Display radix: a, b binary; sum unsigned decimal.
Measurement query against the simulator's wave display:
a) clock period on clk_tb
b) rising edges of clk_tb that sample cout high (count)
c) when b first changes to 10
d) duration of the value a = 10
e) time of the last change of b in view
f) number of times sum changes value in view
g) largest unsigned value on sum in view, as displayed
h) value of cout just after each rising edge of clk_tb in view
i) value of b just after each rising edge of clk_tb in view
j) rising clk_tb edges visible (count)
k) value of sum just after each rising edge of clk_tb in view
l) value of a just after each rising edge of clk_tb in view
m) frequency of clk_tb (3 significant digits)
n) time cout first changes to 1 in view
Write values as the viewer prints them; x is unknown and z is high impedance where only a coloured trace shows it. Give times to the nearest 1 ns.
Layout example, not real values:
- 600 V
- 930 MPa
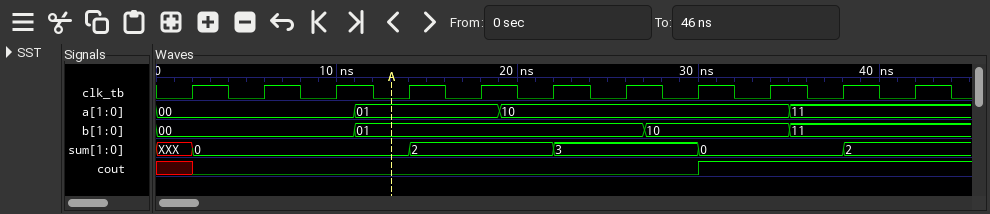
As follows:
- 4 ns
- 3
- 27 ns
- 16 ns
- 35 ns
- 5
- 3
- 0 0 0 0 0 0 0 1 1 1 1
- 00, 00, 00, 01, 01, 01, 01, 10, 10, 11, 11
- 11
- 0, 0, 0, 2, 2, 3, 3, 0, 0, 2, 2
- 00, 00, 00, 01, 01, 10, 10, 10, 10, 11, 11
- 250 MHz
- 30 ns
